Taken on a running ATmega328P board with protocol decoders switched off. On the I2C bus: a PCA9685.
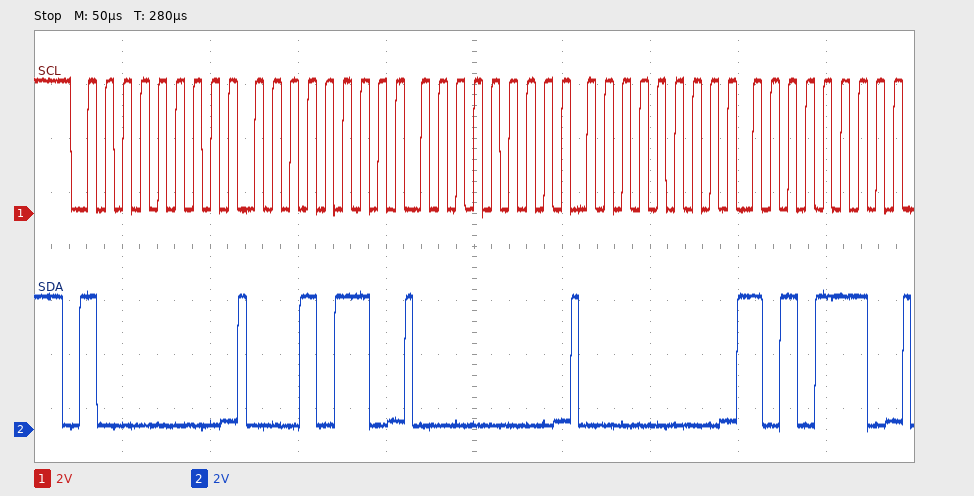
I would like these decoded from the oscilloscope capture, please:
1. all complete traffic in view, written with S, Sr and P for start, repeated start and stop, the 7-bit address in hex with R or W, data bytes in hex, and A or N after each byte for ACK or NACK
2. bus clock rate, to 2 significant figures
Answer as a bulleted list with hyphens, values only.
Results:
- S 40W A 16 A 00 A 00 A AE A
- 100 kHz
